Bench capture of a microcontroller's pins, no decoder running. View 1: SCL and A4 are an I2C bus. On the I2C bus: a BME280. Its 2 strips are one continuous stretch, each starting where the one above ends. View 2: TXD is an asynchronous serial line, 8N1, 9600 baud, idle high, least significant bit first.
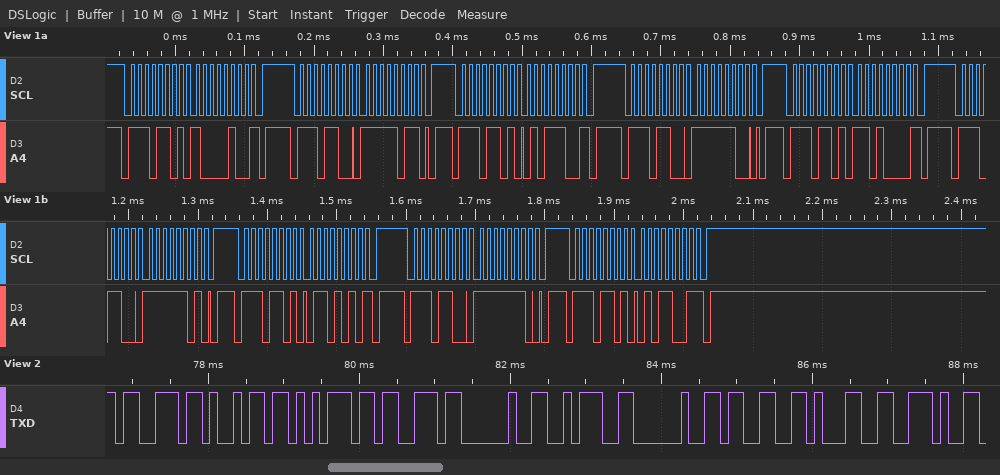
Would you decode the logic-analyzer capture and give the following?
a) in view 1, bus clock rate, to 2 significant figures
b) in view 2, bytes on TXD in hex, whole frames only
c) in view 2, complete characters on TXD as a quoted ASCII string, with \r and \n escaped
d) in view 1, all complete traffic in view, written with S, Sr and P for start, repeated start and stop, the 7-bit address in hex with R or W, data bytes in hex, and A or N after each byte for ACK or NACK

100 kHz
73 69 75 73 20 3A 20 33 31 2E
"sius : 31."
S 76R A 84 N P S 76W A FB A P S 76R A 5C N P S 76W A FC A P S 76R A D0 N P S 76W A FD A P S 76R A 6A N P S 76W A FE A P S 76R A 59 N P
